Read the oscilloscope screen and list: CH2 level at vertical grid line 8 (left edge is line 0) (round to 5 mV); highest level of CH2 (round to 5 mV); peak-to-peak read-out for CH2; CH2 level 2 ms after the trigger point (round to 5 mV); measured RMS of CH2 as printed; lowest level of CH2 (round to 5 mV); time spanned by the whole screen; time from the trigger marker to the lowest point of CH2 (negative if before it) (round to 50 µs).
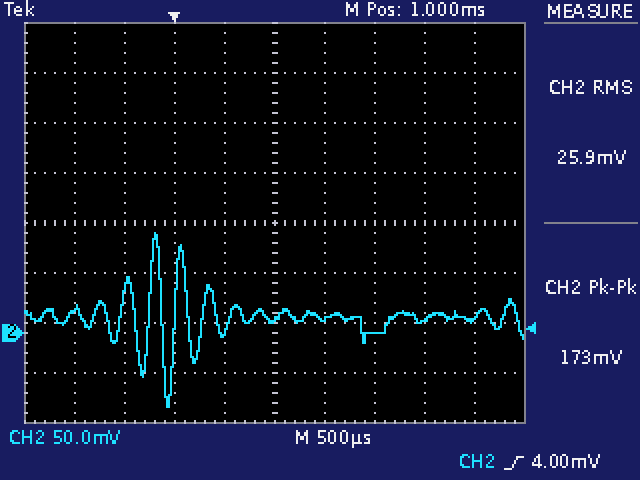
15 mV
100 mV
173 mV
0 mV
25.9 mV
-75 mV
5 ms
-50 µs
